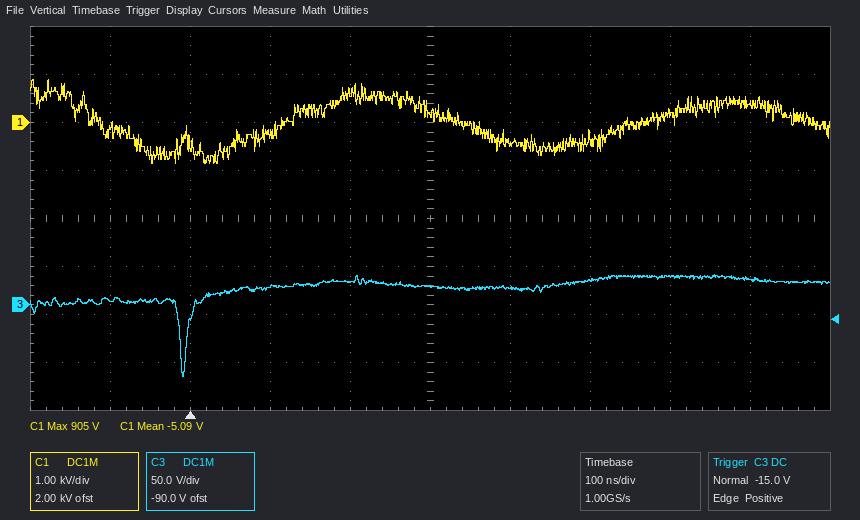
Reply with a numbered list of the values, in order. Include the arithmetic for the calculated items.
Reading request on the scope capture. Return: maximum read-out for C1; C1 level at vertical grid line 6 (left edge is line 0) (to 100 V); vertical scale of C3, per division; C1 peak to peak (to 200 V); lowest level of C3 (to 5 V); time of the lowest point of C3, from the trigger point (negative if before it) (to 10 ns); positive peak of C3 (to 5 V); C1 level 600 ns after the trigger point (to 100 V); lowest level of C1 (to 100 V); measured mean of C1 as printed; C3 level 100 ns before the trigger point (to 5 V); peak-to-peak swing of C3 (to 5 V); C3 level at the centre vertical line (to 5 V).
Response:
1. 905 V
2. -400 V
3. 50 V
4. 1.8 kV
5. -75 V
6. -10 ns
7. 30 V
8. 200 V
9. -900 V
10. -5.09 V
11. 5 V
12. 30 V − (-75 V) = 105 V
13. 20 V
